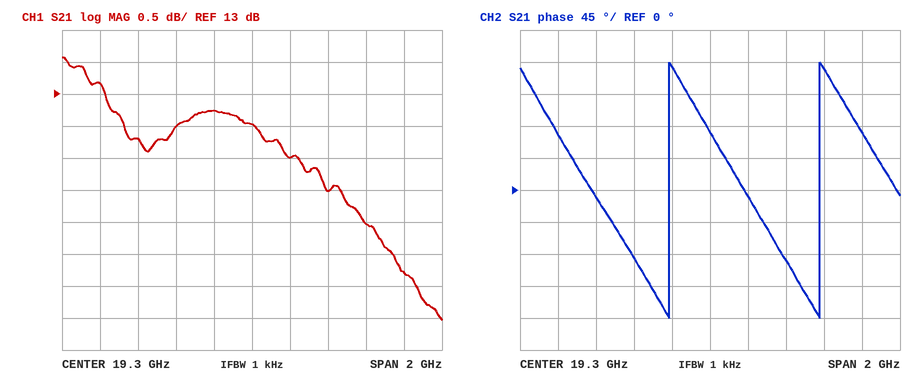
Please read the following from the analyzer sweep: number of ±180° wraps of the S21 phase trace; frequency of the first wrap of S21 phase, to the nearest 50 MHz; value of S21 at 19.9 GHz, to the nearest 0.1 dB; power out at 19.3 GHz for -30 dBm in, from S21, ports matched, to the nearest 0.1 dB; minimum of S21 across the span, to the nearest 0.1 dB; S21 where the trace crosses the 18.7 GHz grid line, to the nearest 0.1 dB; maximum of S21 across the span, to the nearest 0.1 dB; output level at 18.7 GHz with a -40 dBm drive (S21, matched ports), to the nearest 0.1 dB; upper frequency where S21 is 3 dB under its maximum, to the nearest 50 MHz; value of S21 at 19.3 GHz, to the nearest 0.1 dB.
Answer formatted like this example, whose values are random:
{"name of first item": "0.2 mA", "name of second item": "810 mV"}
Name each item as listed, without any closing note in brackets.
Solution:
{"number of ±180° wraps of the S21 phase trace": "2", "frequency of the first wrap of S21 phase, to the nearest 50 MHz": "19.10 GHz", "value of S21 at 19.9 GHz, to the nearest 0.1 dB": "11.0 dB", "power out at 19.3 GHz for -30 dBm in, from S21, ports matched, to the nearest 0.1 dB": "-17.5 dBm", "minimum of S21 across the span, to the nearest 0.1 dB": "9.5 dB", "S21 where the trace crosses the 18.7 GHz grid line, to the nearest 0.1 dB": "12.3 dB", "maximum of S21 across the span, to the nearest 0.1 dB": "13.6 dB", "output level at 18.7 GHz with a -40 dBm drive (S21, matched ports), to the nearest 0.1 dB": "-27.7 dBm", "upper frequency where S21 is 3 dB under its maximum, to the nearest 50 MHz": "20.00 GHz", "value of S21 at 19.3 GHz, to the nearest 0.1 dB": "12.5 dB"}
